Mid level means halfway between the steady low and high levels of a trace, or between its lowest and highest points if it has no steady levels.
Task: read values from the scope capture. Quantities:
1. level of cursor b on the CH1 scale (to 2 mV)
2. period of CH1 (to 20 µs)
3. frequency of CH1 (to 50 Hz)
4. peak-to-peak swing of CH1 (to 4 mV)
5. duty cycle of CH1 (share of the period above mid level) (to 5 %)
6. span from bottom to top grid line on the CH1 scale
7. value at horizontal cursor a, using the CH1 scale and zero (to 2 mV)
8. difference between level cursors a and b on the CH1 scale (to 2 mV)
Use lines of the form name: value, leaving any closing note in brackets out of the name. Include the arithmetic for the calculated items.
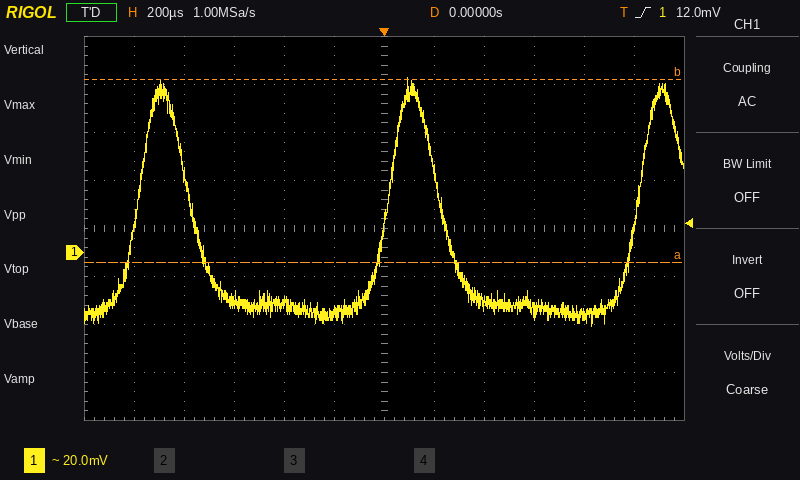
level of cursor b on the CH1 scale: 72 mV
period of CH1: 1.00 ms
frequency of CH1: 1 / 1.00 ms ≈ 1.00 kHz
peak-to-peak swing of CH1: 104 mV
duty cycle of CH1 (share of the period above mid level): 20 %
span from bottom to top grid line on the CH1 scale: 160 mV
value at horizontal cursor a, using the CH1 scale and zero: -4 mV
difference between level cursors a and b on the CH1 scale: 76 mV
